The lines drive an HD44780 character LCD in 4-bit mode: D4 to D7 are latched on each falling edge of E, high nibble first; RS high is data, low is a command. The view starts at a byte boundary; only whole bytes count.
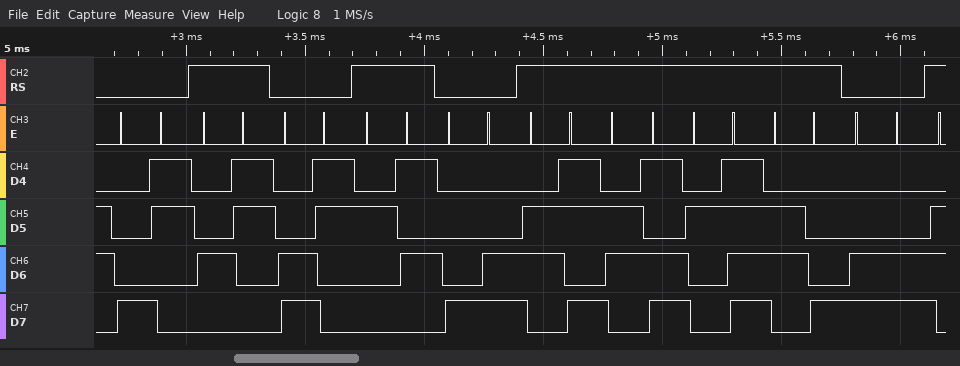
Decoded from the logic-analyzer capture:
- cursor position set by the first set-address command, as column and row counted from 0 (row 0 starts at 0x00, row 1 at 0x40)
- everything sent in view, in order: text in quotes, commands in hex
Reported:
column 3, row 0
0x83 "C" 0xC3 "%" 0x8C "km/h" 0xCC
